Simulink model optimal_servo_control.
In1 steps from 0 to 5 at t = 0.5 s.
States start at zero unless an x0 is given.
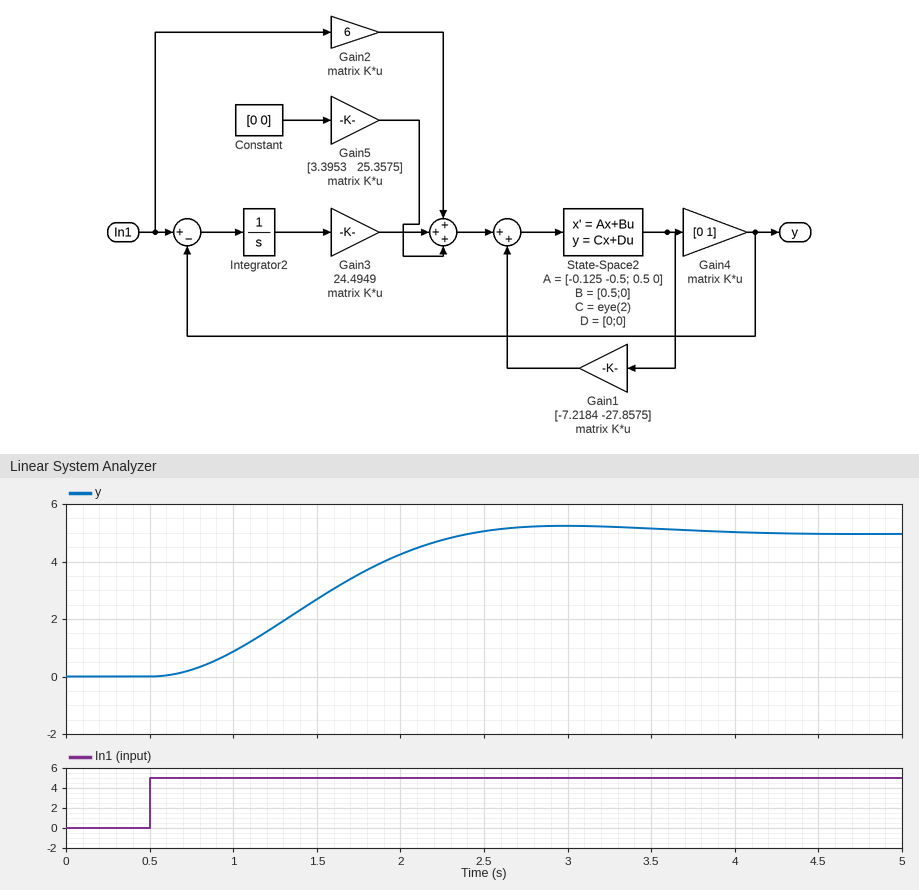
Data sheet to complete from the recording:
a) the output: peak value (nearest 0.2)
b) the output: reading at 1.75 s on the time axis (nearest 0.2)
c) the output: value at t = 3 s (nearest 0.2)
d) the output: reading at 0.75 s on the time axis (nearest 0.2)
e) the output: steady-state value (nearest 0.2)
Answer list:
5.2
3.6
5.2
0.2
5.0
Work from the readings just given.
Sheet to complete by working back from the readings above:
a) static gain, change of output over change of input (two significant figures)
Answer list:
1.0
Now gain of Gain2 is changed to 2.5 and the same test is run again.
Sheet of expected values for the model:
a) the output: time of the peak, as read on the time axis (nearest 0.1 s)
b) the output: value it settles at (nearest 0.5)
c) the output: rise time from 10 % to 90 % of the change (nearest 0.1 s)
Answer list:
3.2 s
5.0
1.3 s
